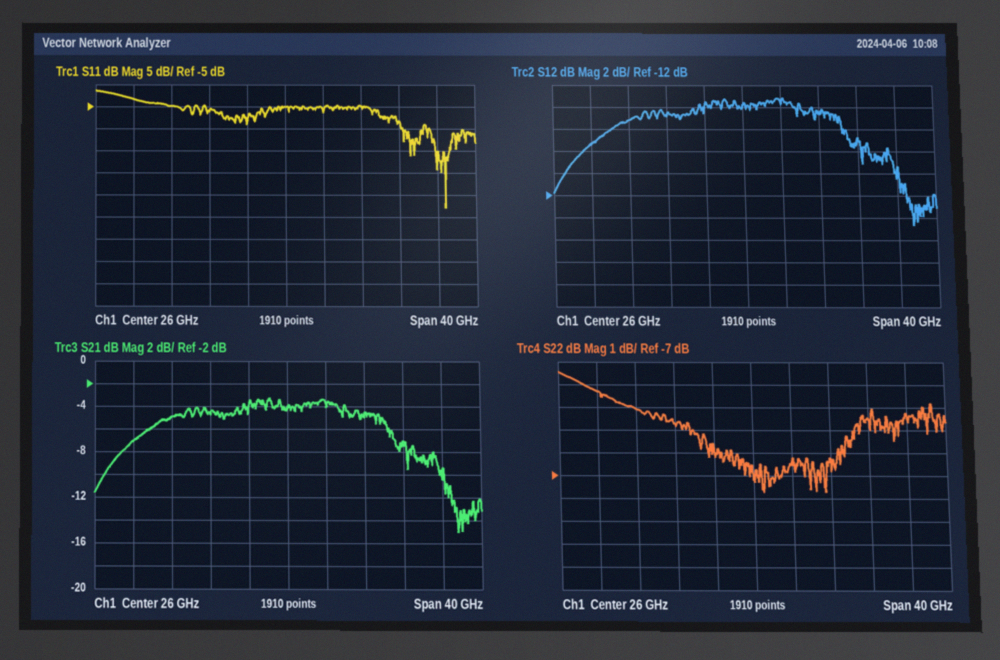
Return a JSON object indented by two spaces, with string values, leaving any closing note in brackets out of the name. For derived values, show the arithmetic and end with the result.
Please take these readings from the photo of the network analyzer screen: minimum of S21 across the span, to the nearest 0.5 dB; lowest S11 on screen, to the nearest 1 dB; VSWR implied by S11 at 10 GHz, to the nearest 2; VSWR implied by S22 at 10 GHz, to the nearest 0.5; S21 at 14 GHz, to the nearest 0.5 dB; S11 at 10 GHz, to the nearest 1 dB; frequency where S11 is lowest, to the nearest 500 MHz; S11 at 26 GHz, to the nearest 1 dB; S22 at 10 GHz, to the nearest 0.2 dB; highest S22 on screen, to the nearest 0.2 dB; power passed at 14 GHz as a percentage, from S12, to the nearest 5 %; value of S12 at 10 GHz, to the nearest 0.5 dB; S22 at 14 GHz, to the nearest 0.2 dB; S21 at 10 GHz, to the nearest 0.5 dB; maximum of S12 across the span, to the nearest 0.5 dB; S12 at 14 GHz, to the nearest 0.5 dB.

{
  "minimum of S21 across the span, to the nearest 0.5 dB": "-15.0 dB",
  "lowest S11 on screen, to the nearest 1 dB": "-28 dB",
  "VSWR implied by S11 at 10 GHz, to the nearest 2": "|Γ| = 10^(-3/20) = 0.7079; VSWR = (1 + 0.7079)/(1 − 0.7079) ≈ 6",
  "VSWR implied by S22 at 10 GHz, to the nearest 0.5": "|Γ| = 10^(-3.2/20) = 0.6918; VSWR = (1 + 0.6918)/(1 − 0.6918) ≈ 5.5",
  "S21 at 14 GHz, to the nearest 0.5 dB": "-5.0 dB",
  "S11 at 10 GHz, to the nearest 1 dB": "-3 dB",
  "frequency where S11 is lowest, to the nearest 500 MHz": "43.0 GHz",
  "S11 at 26 GHz, to the nearest 1 dB": "-5 dB",
  "S22 at 10 GHz, to the nearest 0.2 dB": "-3.2 dB",
  "highest S22 on screen, to the nearest 0.2 dB": "-2.4 dB",
  "power passed at 14 GHz as a percentage, from S12, to the nearest 5 %": "10^(-5/10) ≈ 31.6 %, so 30 % to the nearest 5 %",
  "value of S12 at 10 GHz, to the nearest 0.5 dB": "-7.5 dB",
  "S22 at 14 GHz, to the nearest 0.2 dB": "-4.0 dB",
  "S21 at 10 GHz, to the nearest 0.5 dB": "-7.0 dB",
  "maximum of S12 across the span, to the nearest 0.5 dB": "-3.0 dB",
  "S12 at 14 GHz, to the nearest 0.5 dB": "-5.0 dB"
}
